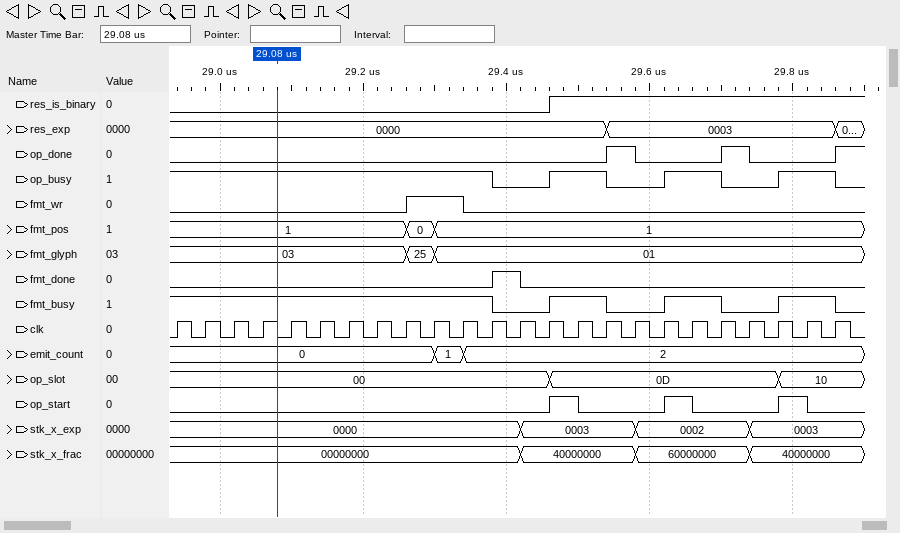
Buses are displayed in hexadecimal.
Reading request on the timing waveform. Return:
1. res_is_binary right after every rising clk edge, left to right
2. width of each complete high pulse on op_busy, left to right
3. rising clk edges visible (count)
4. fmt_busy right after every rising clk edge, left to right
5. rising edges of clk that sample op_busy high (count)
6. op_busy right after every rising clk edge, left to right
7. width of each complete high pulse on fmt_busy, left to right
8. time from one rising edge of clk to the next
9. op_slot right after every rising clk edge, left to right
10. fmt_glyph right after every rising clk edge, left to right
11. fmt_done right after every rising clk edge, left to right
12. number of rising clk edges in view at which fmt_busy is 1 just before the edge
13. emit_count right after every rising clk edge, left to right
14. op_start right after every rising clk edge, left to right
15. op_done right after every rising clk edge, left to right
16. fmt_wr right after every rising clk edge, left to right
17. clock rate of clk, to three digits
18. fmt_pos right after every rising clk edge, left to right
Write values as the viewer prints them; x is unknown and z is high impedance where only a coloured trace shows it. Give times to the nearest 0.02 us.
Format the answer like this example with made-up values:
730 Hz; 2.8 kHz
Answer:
0 0 0 0 0 0 0 0 0 0 0 0 0 1 1 1 1 1 1 1 1 1 1 1; 0.08 us, 0.08 us, 0.08 us; 24; 1 1 1 1 1 1 1 1 1 1 1 0 0 1 1 0 0 1 1 0 0 1 1 0; 18; 1 1 1 1 1 1 1 1 1 1 1 0 0 1 1 0 0 1 1 0 0 1 1 0; 0.08 us, 0.08 us, 0.08 us; 0.04 us; 00, 00, 00, 00, 00, 00, 00, 00, 00, 00, 00, 00, 00, 0D, 0D, 0D, 0D, 0D, 0D, 0D, 0D, 10, 10, 10; 03, 03, 03, 03, 03, 03, 03, 03, 25, 01, 01, 01, 01, 01, 01, 01, 01, 01, 01, 01, 01, 01, 01, 01; 0 0 0 0 0 0 0 0 0 0 0 1 0 0 0 0 0 0 0 0 0 0 0 0; 18; 0, 0, 0, 0, 0, 0, 0, 0, 0, 1, 2, 2, 2, 2, 2, 2, 2, 2, 2, 2, 2, 2, 2, 2; 0 0 0 0 0 0 0 0 0 0 0 0 0 1 0 0 0 1 0 0 0 1 0 0; 0 0 0 0 0 0 0 0 0 0 0 0 0 0 0 1 0 0 0 1 0 0 0 1; 0 0 0 0 0 0 0 0 1 1 0 0 0 0 0 0 0 0 0 0 0 0 0 0; 25.0 MHz; 1, 1, 1, 1, 1, 1, 1, 1, 0, 1, 1, 1, 1, 1, 1, 1, 1, 1, 1, 1, 1, 1, 1, 1
